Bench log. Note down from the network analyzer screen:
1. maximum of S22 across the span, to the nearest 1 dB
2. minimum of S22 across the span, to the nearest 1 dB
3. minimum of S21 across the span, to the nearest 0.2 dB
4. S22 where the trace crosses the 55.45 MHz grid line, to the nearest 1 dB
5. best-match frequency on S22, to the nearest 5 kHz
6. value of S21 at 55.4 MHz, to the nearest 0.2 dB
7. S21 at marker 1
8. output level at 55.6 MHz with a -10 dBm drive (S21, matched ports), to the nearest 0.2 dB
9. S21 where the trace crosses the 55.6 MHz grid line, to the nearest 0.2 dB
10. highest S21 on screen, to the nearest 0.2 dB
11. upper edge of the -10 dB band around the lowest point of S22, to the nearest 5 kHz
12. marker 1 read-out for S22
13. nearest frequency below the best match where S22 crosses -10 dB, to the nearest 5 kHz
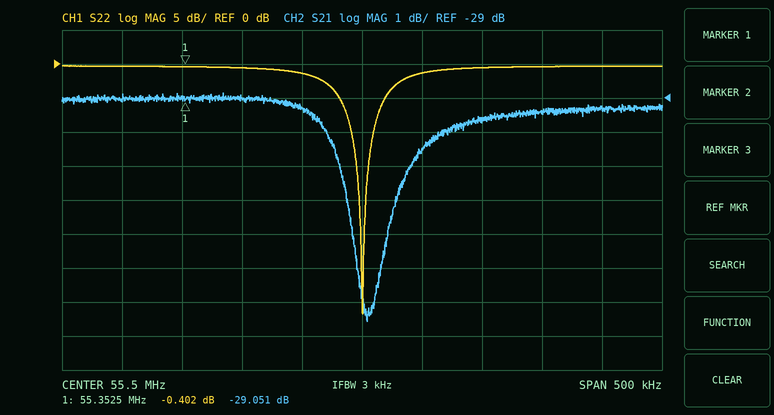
0 dB
-37 dB
-35.6 dB
-1 dB
55.500 MHz
-29.0 dB
-29.051 dB
-39.6 dBm
-29.6 dB
-28.8 dB
55.510 MHz
-0.402 dB
55.490 MHz
